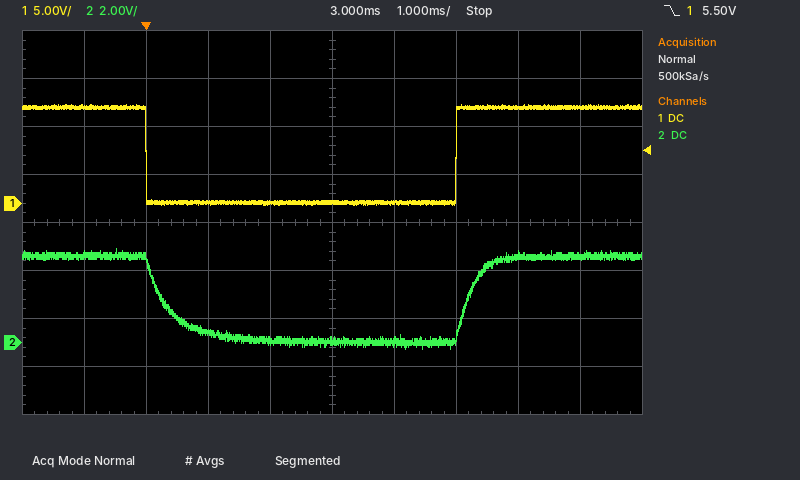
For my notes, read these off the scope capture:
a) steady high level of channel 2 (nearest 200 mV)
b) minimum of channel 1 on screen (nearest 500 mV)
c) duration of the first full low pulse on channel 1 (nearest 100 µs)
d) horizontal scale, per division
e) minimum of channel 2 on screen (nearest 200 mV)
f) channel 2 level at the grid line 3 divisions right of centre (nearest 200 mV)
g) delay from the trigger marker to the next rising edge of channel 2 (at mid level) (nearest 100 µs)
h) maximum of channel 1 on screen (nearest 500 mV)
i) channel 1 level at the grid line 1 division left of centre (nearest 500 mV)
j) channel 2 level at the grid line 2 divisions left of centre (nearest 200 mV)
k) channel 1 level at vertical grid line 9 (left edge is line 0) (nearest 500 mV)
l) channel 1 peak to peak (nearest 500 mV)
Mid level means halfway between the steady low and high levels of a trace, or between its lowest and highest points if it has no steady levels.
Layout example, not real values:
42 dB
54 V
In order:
3.6 V
0.0 V
5.0 ms
1 ms
-200 mV
3.6 V
5.2 ms
10.5 V
0.0 V
400 mV
10.0 V
10.5 V
